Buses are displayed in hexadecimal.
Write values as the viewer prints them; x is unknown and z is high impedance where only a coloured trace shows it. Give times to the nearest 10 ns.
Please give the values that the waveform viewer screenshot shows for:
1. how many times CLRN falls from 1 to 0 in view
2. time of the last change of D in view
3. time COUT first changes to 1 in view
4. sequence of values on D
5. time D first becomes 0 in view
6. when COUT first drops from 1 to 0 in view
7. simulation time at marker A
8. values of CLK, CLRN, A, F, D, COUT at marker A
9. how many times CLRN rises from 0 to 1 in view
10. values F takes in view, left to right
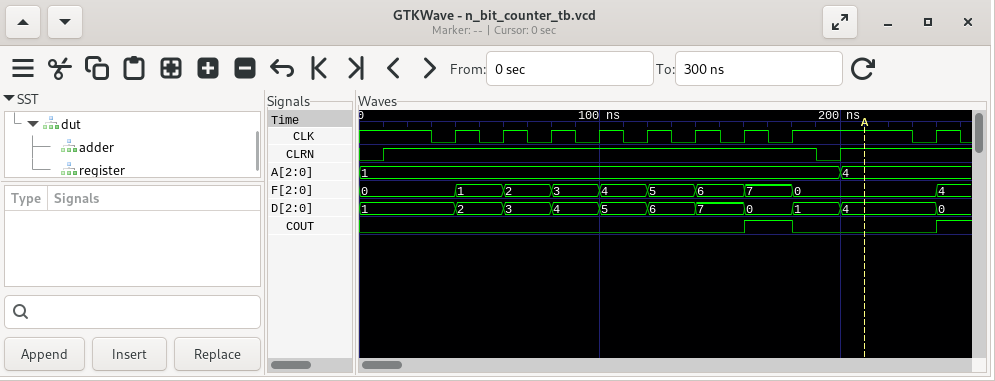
1
240 ns
160 ns
1, 2, 3, 4, 5, 6, 7, 0, 1, 4, 0
160 ns
180 ns
210 ns
CLK=1, CLRN=1, A=4, F=0, D=4, COUT=0
2
0, 1, 2, 3, 4, 5, 6, 7, 0, 4
